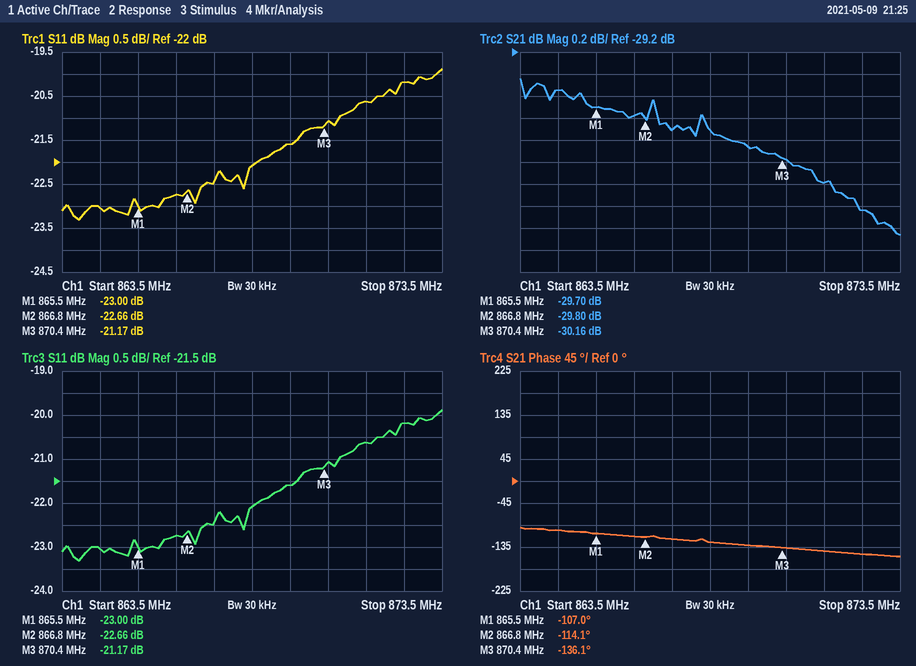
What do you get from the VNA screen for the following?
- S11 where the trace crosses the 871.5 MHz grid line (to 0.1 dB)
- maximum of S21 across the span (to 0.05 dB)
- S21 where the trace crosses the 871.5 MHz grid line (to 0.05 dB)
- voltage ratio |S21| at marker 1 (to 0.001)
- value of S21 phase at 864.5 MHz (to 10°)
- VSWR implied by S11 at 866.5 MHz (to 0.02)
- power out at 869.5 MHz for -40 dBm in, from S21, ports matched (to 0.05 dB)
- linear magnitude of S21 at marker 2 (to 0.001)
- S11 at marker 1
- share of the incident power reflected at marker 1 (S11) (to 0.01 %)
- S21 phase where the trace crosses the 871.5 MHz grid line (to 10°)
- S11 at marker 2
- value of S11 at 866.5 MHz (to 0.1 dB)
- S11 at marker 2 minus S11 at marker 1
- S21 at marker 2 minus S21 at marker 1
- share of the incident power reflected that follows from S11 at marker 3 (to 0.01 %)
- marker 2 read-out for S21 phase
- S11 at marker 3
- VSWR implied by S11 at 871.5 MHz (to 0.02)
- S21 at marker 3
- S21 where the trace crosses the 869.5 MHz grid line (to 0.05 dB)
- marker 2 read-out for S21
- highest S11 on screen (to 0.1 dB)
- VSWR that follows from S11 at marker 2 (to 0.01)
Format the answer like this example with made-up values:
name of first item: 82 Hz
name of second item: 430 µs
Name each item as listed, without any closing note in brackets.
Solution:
S11 where the trace crosses the 871.5 MHz grid line: -20.6 dB
maximum of S21 across the span: -29.45 dB
S21 where the trace crosses the 871.5 MHz grid line: -30.40 dB
voltage ratio |S21| at marker 1: 0.033
value of S21 phase at 864.5 MHz: -100°
VSWR implied by S11 at 866.5 MHz: 1.16
power out at 869.5 MHz for -40 dBm in, from S21, ports matched: -70.05 dBm
linear magnitude of S21 at marker 2: 0.032
S11 at marker 1: -23.00 dB
share of the incident power reflected at marker 1 (S11): 0.50 %
S21 phase where the trace crosses the 871.5 MHz grid line: -140°
S11 at marker 2: -22.66 dB
value of S11 at 866.5 MHz: -22.7 dB
S11 at marker 2 minus S11 at marker 1: 0.34 dB
S21 at marker 2 minus S21 at marker 1: -0.10 dB
share of the incident power reflected that follows from S11 at marker 3: 0.76 %
marker 2 read-out for S21 phase: -114.1°
S11 at marker 3: -21.17 dB
VSWR implied by S11 at 871.5 MHz: 1.20
S21 at marker 3: -30.16 dB
S21 where the trace crosses the 869.5 MHz grid line: -30.05 dB
marker 2 read-out for S21: -29.80 dB
highest S11 on screen: -19.9 dB
VSWR that follows from S11 at marker 2: 1.16
